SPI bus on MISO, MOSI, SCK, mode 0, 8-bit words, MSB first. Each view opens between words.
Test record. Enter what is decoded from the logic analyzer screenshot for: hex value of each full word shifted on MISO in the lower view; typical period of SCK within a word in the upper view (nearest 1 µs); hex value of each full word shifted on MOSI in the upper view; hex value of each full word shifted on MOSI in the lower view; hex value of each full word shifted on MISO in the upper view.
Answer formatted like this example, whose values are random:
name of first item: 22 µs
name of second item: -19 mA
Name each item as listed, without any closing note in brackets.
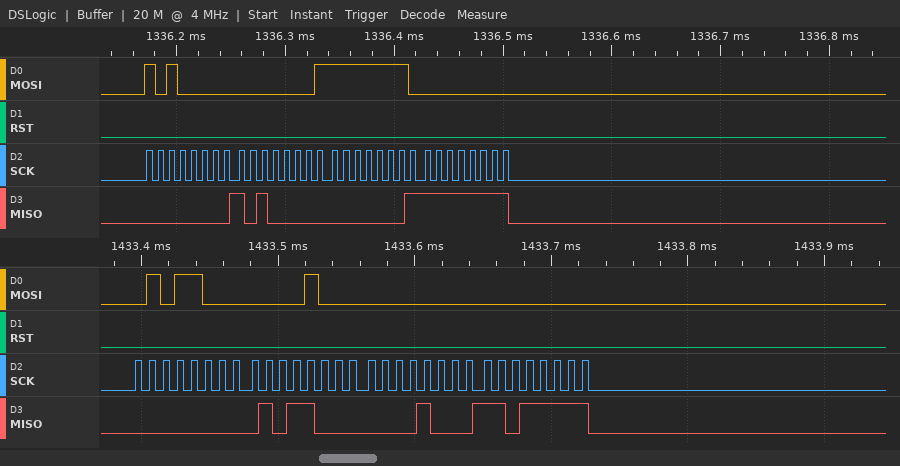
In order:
hex value of each full word shifted on MISO in the lower view: 00, 58, 08, DF
typical period of SCK within a word in the upper view: 10 µs
hex value of each full word shifted on MOSI in the upper view: A0, 01, FE, 00
hex value of each full word shifted on MOSI in the lower view: 58, 08, 00, 00
hex value of each full word shifted on MISO in the upper view: 00, A0, 01, FF
